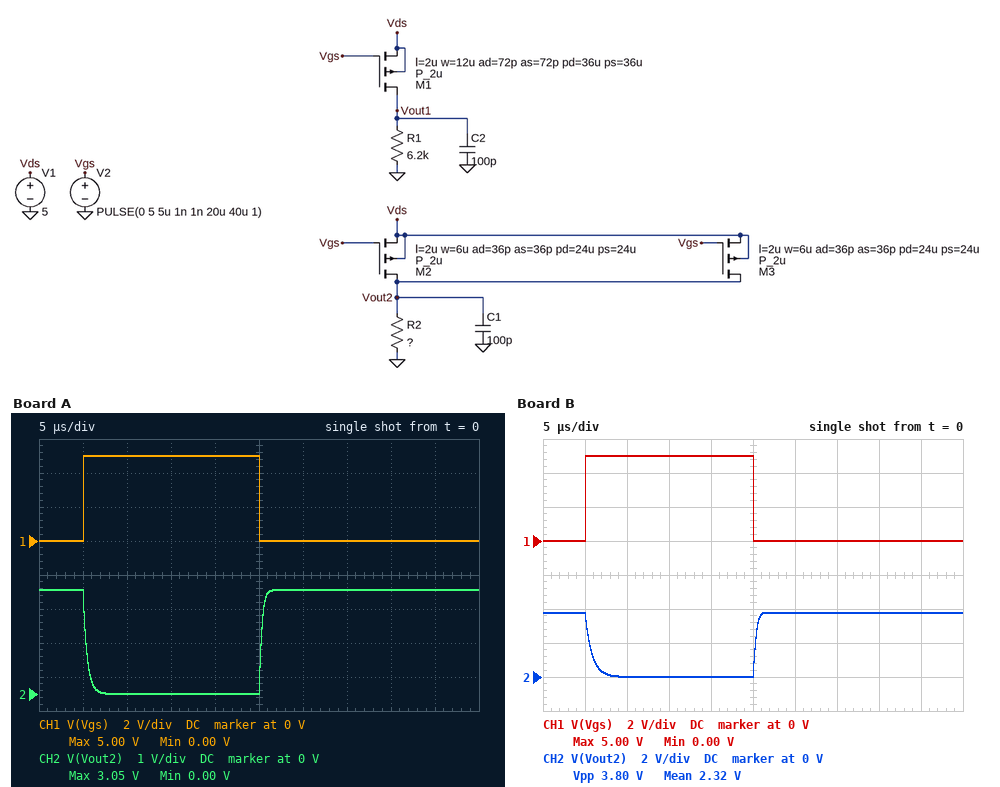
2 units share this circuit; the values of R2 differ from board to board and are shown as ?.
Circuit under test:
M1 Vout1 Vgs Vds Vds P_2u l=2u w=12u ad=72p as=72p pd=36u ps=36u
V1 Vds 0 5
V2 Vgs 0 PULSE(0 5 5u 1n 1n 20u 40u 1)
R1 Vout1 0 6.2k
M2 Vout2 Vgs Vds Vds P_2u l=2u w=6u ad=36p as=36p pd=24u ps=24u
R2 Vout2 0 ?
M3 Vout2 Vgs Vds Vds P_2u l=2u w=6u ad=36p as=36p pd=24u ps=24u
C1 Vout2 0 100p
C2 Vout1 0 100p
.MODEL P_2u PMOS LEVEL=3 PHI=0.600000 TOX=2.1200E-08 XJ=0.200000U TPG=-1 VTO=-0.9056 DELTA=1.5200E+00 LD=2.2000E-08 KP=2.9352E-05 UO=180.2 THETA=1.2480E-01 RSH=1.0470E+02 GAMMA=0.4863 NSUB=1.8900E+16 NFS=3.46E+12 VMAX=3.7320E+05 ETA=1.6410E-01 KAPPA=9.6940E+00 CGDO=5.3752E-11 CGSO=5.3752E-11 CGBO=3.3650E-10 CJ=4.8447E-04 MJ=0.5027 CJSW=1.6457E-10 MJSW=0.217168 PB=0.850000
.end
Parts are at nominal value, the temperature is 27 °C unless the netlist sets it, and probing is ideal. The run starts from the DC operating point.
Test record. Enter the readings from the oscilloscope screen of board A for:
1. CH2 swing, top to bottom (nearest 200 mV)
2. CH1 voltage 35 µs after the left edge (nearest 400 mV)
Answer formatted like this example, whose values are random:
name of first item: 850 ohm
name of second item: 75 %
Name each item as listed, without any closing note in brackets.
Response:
CH2 swing, top to bottom: 3.0 V
CH1 voltage 35 µs after the left edge: 0 V
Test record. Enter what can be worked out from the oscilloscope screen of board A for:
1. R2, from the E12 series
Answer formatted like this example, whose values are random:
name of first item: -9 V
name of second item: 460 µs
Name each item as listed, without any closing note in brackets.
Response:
R2, from the E12 series: 4.7 kΩ
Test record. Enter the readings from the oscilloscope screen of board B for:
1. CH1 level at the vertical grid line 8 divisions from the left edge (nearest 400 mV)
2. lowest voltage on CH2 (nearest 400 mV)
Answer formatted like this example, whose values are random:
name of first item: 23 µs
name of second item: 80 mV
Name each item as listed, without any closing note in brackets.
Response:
CH1 level at the vertical grid line 8 divisions from the left edge: 0 V
lowest voltage on CH2: 0 V
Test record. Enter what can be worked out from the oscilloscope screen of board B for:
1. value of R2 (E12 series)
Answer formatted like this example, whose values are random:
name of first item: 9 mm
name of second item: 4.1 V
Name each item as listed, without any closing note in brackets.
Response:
value of R2: 8.2 kΩ
